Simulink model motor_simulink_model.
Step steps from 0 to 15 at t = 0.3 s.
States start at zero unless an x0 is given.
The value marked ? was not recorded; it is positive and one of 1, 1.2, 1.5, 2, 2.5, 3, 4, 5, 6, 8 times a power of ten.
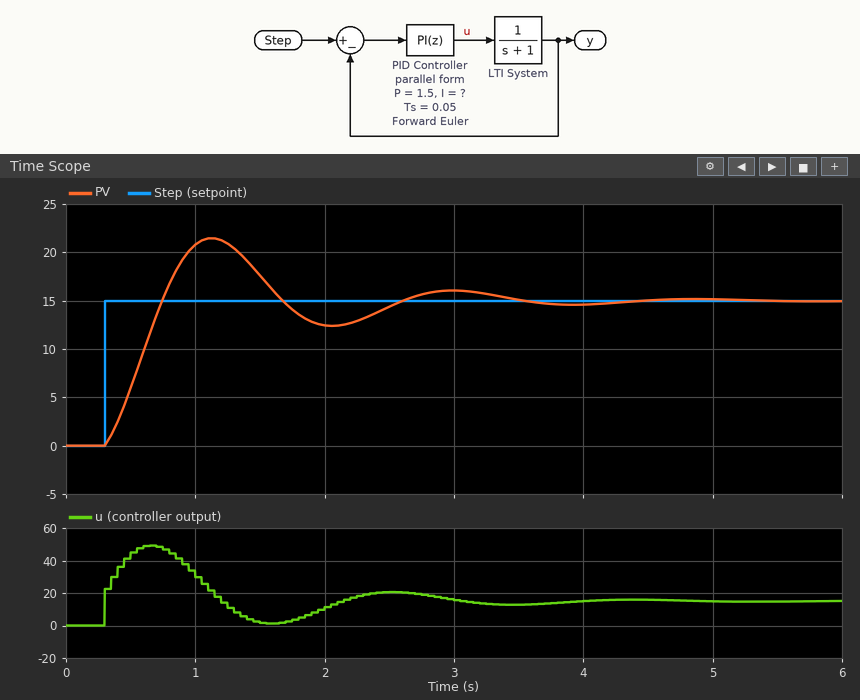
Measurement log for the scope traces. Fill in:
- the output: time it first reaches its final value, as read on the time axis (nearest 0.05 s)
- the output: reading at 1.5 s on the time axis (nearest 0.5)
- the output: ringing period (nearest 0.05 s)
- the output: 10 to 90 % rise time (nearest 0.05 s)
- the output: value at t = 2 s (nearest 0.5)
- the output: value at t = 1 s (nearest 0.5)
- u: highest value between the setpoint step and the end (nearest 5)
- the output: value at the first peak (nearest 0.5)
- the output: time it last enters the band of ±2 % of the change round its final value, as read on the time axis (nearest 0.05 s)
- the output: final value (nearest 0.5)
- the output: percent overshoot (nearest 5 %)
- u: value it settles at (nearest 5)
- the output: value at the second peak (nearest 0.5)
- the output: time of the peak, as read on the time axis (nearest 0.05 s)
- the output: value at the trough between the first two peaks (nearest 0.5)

0.75 s
17.5
1.85 s
0.35 s
12.5
21.0
50
21.5
4.15 s
15.0
45 %
15
16.0
1.15 s
12.5
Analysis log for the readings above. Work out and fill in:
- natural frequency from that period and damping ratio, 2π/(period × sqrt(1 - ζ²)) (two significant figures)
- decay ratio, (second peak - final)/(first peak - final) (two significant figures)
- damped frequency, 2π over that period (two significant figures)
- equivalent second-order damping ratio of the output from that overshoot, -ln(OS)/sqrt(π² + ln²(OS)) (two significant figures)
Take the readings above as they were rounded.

3.5 rad/s
0.15
3.4 rad/s
0.25
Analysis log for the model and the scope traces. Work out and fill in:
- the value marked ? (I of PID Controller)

12
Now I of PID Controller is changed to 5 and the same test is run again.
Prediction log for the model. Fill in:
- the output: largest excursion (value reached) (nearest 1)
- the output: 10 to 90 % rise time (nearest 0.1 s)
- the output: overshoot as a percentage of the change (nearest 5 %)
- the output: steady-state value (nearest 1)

18
0.6 s
20 %
15
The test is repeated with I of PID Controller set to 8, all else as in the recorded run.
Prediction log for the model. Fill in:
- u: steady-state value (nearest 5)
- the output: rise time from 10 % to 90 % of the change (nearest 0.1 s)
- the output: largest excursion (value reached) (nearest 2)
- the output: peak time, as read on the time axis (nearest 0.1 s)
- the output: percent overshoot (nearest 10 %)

15
0.4 s
20
1.3 s
30 %
